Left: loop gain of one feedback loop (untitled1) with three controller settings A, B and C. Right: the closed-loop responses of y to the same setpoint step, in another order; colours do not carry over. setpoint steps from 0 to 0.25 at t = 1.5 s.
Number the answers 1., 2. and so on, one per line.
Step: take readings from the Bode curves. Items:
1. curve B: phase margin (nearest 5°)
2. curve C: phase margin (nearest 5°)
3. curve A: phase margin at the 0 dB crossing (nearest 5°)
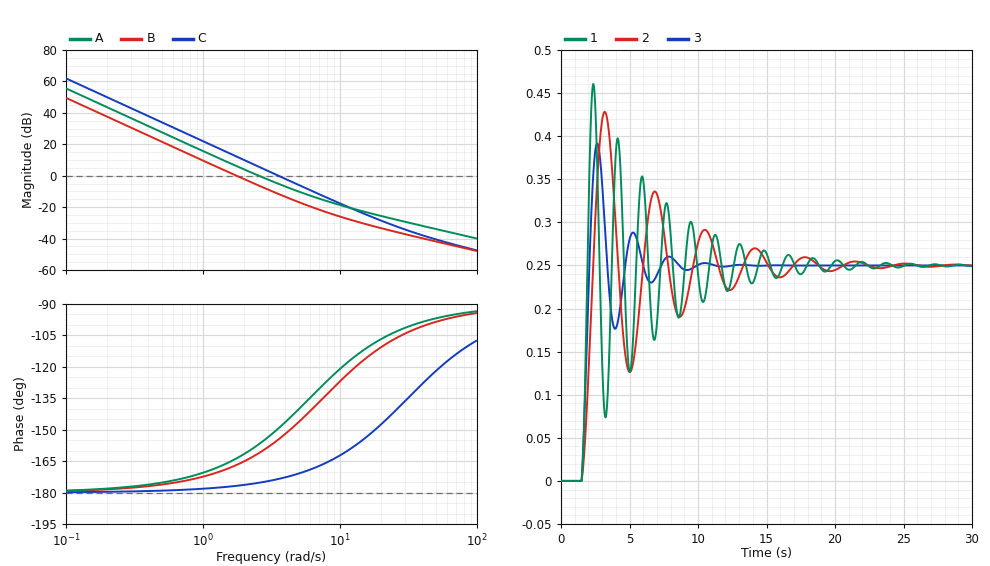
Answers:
1. 15°
2. 5°
3. 25°
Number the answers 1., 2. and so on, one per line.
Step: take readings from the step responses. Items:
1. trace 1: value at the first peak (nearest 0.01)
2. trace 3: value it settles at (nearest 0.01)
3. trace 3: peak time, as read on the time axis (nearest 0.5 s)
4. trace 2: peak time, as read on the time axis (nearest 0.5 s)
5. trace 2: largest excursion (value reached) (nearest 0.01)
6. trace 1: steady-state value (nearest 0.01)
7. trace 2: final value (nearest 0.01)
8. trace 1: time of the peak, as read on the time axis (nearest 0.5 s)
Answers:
1. 0.46
2. 0.25
3. 2.5 s
4. 3.0 s
5. 0.43
6. 0.25
7. 0.25
8. 2.5 s
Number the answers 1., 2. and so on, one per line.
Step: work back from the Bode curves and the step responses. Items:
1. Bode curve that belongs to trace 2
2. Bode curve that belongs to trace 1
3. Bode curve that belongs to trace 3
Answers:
1. B
2. C
3. A
